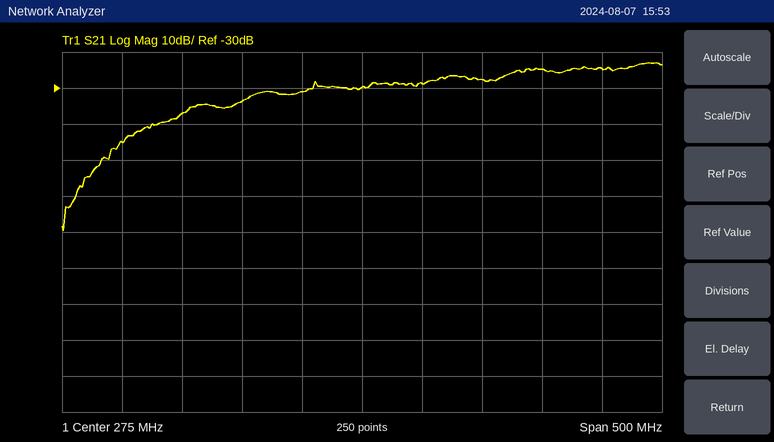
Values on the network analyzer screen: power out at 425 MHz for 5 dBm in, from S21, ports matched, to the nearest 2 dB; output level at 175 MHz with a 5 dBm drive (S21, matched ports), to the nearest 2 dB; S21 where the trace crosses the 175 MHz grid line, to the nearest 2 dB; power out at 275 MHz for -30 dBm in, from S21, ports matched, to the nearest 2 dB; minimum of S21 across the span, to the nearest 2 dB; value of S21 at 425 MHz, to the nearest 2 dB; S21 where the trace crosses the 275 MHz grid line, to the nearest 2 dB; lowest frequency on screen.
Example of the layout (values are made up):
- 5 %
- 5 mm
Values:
- -20 dBm
- -28 dBm
- -34 dB
- -60 dBm
- -70 dB
- -24 dB
- -30 dB
- 25 MHz
